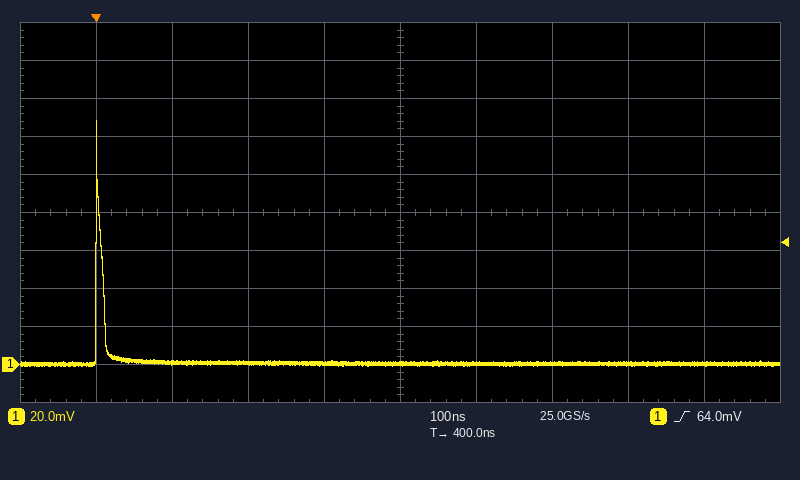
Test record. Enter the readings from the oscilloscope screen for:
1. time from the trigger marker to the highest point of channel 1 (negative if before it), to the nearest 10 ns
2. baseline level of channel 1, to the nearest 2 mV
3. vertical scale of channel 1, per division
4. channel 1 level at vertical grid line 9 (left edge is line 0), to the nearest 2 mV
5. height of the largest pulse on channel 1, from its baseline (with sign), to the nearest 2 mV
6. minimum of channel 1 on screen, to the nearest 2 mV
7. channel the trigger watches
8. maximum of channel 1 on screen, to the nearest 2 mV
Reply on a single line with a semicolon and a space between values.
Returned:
0 ns; 0 mV; 20 mV; 0 mV; +128 mV; 0 mV; channel 1; 128 mV
